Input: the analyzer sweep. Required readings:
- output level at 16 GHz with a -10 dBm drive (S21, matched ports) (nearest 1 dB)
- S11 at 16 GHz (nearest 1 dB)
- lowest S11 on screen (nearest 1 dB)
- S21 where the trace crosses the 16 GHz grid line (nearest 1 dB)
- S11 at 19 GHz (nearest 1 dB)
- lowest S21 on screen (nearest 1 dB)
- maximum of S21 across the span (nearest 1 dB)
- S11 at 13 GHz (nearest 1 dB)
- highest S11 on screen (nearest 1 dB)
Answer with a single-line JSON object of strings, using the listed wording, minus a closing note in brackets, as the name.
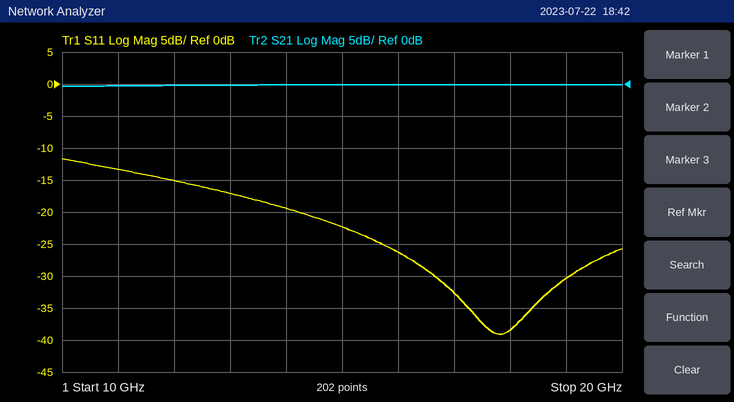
{"output level at 16 GHz with a -10 dBm drive (S21, matched ports)": "-10 dBm", "S11 at 16 GHz": "-26 dB", "lowest S11 on screen": "-39 dB", "S21 where the trace crosses the 16 GHz grid line": "0 dB", "S11 at 19 GHz": "-30 dB", "lowest S21 on screen": "0 dB", "maximum of S21 across the span": "0 dB", "S11 at 13 GHz": "-17 dB", "highest S11 on screen": "-12 dB"}
